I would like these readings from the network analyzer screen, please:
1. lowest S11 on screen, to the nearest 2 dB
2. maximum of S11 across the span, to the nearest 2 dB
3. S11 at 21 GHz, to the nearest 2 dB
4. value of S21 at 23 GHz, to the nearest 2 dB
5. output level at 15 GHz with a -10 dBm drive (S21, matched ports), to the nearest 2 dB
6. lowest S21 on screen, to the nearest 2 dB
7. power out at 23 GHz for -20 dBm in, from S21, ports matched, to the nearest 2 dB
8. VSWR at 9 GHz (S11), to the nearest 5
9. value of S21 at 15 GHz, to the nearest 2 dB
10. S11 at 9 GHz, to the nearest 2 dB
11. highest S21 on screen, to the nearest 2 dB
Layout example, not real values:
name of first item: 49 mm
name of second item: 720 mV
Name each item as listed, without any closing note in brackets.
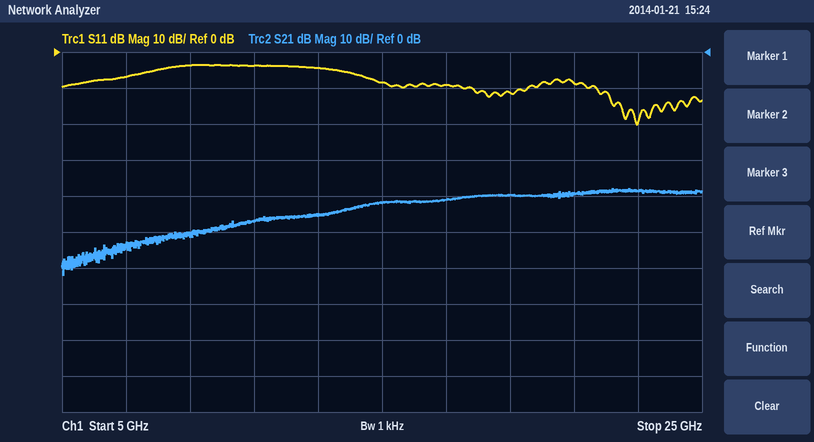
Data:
lowest S11 on screen, to the nearest 2 dB: -20 dB
maximum of S11 across the span, to the nearest 2 dB: -4 dB
S11 at 21 GHz, to the nearest 2 dB: -8 dB
value of S21 at 23 GHz, to the nearest 2 dB: -38 dB
output level at 15 GHz with a -10 dBm drive (S21, matched ports), to the nearest 2 dB: -52 dBm
lowest S21 on screen, to the nearest 2 dB: -62 dB
power out at 23 GHz for -20 dBm in, from S21, ports matched, to the nearest 2 dB: -58 dBm
VSWR at 9 GHz (S11), to the nearest 5: 5
value of S21 at 15 GHz, to the nearest 2 dB: -42 dB
S11 at 9 GHz, to the nearest 2 dB: -4 dB
highest S21 on screen, to the nearest 2 dB: -38 dB
